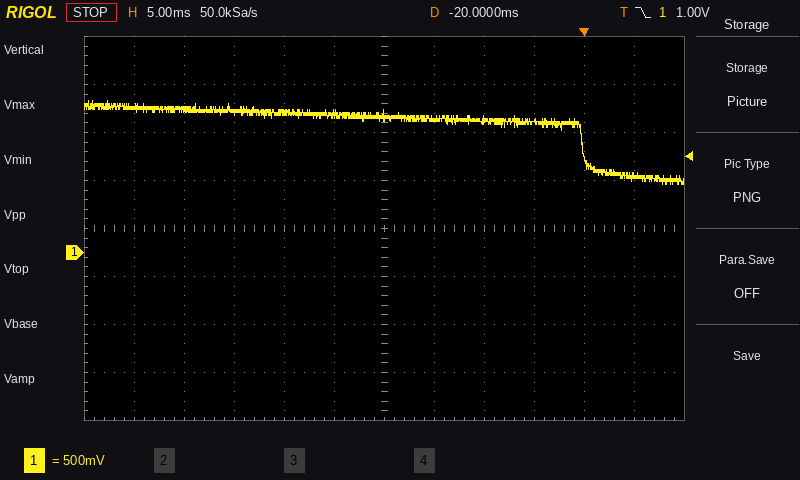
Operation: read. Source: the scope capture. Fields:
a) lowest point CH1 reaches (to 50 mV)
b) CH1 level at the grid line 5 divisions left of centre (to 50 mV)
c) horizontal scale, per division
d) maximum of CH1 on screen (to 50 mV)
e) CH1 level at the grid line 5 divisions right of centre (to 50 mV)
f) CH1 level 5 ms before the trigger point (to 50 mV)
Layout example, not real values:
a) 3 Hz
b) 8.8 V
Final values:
a) 700 mV
b) 1.50 V
c) 5 ms
d) 1.60 V
e) 800 mV
f) 1.35 V
